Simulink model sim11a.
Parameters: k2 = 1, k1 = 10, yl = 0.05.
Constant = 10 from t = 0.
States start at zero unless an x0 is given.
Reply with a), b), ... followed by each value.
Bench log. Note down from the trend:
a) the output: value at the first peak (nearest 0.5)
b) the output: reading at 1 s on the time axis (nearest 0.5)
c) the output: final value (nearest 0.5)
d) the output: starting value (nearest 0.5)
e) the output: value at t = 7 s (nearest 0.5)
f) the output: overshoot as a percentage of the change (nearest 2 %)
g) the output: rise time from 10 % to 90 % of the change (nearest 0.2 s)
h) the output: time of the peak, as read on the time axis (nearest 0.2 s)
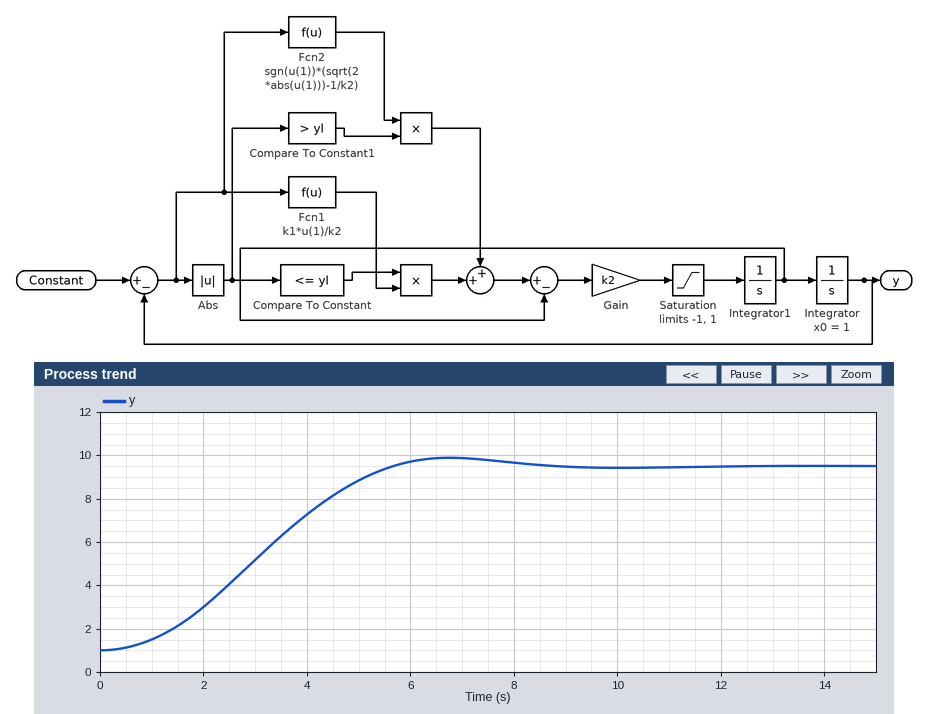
a) 10.0
b) 1.5
c) 9.5
d) 1.0
e) 10.0
f) 4 %
g) 3.6 s
h) 6.8 s
